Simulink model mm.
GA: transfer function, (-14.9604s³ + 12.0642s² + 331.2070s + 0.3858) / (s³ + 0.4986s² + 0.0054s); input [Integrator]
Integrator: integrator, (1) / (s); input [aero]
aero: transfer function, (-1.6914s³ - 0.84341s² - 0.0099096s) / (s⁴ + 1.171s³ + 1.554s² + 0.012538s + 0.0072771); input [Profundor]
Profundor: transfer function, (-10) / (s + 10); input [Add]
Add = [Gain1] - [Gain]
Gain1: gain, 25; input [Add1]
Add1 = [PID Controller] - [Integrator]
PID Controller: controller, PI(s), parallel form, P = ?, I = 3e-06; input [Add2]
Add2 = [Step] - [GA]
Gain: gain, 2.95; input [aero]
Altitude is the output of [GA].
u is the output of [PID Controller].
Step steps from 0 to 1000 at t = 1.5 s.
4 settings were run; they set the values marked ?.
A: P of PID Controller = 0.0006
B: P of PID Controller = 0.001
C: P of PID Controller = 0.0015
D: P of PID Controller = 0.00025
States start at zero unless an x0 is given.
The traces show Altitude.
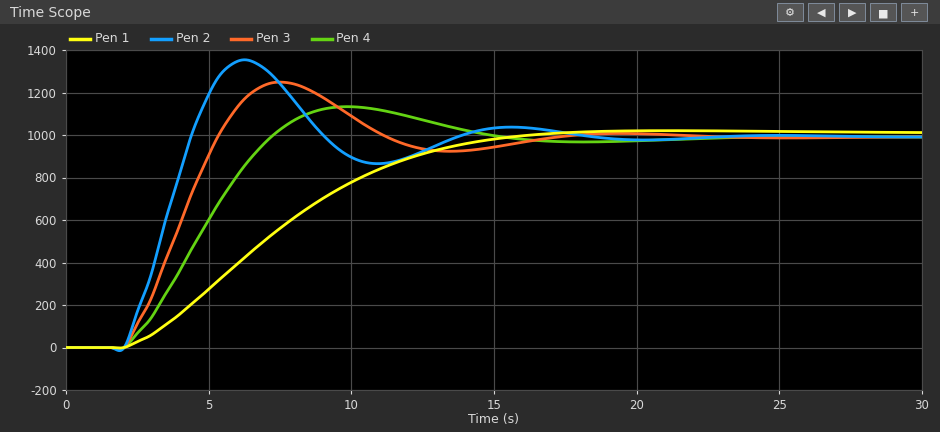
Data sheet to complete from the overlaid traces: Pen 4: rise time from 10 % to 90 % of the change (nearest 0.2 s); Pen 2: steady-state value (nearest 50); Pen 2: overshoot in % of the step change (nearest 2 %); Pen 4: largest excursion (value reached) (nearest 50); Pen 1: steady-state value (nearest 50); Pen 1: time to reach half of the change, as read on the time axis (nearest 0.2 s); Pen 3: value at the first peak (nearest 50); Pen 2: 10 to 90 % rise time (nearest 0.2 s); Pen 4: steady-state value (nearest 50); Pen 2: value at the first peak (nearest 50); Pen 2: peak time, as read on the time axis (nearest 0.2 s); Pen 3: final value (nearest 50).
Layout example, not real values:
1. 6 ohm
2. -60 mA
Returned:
1. 3.8 s
2. 1000
3. 36 %
4. 1150
5. 1000
6. 7.0 s
7. 1250
8. 1.8 s
9. 1000
10. 1350
11. 6.2 s
12. 1000
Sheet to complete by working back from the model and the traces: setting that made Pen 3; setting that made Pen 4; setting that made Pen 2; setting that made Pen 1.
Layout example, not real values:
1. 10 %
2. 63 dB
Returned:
1. B
2. A
3. C
4. D
